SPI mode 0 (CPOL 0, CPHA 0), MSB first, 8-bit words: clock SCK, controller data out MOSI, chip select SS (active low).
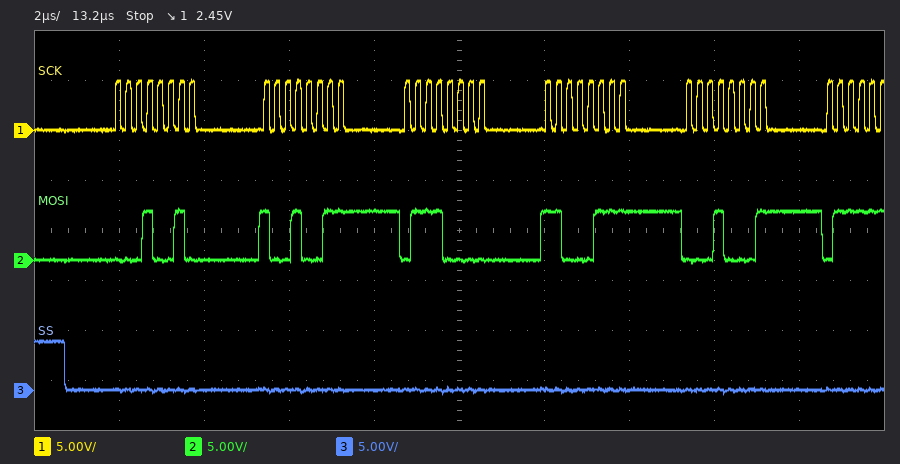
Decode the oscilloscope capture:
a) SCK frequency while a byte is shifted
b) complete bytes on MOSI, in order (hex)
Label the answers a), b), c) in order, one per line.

a) 4 MHz
b) 0x12 0x93 0x70 0xC7 0x11
